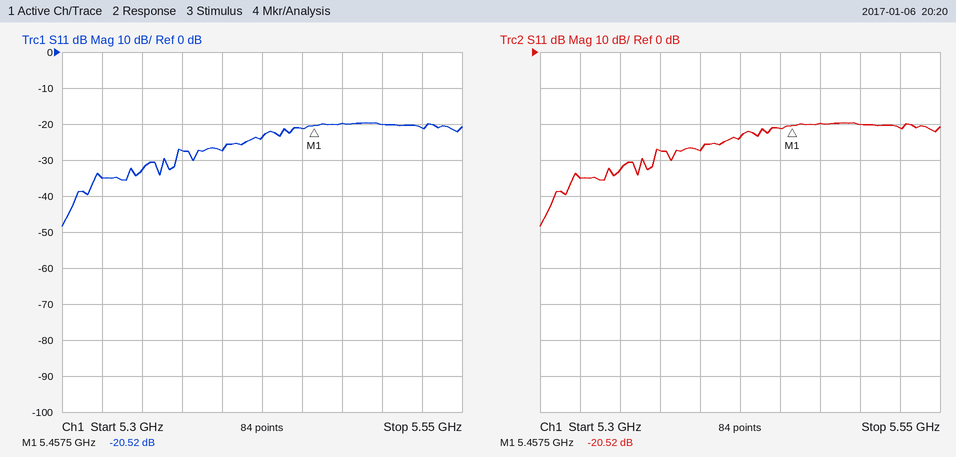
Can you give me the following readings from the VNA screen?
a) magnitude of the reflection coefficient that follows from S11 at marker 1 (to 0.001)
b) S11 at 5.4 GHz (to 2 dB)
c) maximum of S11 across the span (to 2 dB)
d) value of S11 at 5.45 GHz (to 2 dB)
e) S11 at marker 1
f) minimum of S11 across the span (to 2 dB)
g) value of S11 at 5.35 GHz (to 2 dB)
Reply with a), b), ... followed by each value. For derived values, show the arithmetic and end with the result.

a) 10^(-20.52/20) ≈ 0.094
b) -28 dB
c) -20 dB
d) -22 dB
e) -20.52 dB
f) -48 dB
g) -32 dB
